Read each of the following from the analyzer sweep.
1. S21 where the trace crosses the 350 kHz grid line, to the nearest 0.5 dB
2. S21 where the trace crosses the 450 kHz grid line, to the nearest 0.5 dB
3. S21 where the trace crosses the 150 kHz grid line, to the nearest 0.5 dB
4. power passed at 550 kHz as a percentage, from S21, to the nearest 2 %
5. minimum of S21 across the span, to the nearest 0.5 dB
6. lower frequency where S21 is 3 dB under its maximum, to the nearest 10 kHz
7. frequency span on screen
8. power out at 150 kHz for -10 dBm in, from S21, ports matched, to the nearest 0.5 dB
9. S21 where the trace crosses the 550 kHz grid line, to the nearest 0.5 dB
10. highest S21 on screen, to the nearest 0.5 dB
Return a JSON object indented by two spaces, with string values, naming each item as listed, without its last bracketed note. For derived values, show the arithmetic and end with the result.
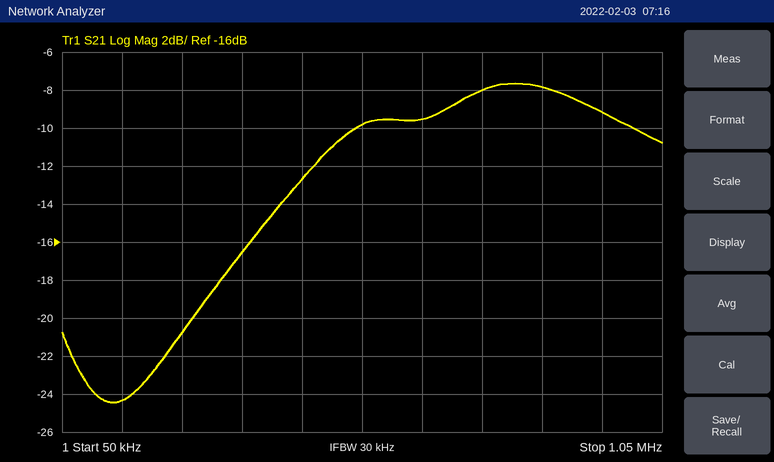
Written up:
{
  "S21 where the trace crosses the 350 kHz grid line, to the nearest 0.5 dB": "-16.5 dB",
  "S21 where the trace crosses the 450 kHz grid line, to the nearest 0.5 dB": "-12.5 dB",
  "S21 where the trace crosses the 150 kHz grid line, to the nearest 0.5 dB": "-24.5 dB",
  "power passed at 550 kHz as a percentage, from S21, to the nearest 2 %": "10^(-10/10) ≈ 10 %",
  "minimum of S21 across the span, to the nearest 0.5 dB": "-24.5 dB",
  "lower frequency where S21 is 3 dB under its maximum, to the nearest 10 kHz": "510 kHz",
  "frequency span on screen": "1 MHz",
  "power out at 150 kHz for -10 dBm in, from S21, ports matched, to the nearest 0.5 dB": "-10 dBm + (-24.5 dB) = -34.5 dBm",
  "S21 where the trace crosses the 550 kHz grid line, to the nearest 0.5 dB": "-10.0 dB",
  "highest S21 on screen, to the nearest 0.5 dB": "-7.5 dB"
}
